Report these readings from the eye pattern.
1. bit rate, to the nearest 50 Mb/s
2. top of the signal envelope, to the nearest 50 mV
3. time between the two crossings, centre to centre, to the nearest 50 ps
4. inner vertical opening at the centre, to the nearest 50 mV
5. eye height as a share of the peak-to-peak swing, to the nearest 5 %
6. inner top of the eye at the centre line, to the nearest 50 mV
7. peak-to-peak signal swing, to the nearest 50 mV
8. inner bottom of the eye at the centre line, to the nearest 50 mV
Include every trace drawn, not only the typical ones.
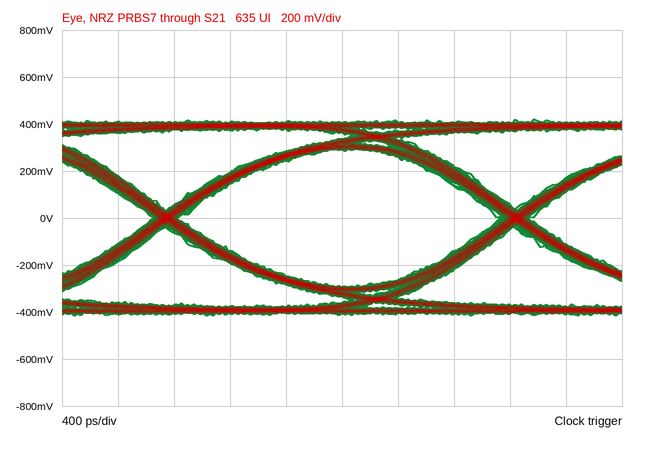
400 Mb/s
400 mV
2.50 ns
600 mV
70 %
300 mV
850 mV
-300 mV
